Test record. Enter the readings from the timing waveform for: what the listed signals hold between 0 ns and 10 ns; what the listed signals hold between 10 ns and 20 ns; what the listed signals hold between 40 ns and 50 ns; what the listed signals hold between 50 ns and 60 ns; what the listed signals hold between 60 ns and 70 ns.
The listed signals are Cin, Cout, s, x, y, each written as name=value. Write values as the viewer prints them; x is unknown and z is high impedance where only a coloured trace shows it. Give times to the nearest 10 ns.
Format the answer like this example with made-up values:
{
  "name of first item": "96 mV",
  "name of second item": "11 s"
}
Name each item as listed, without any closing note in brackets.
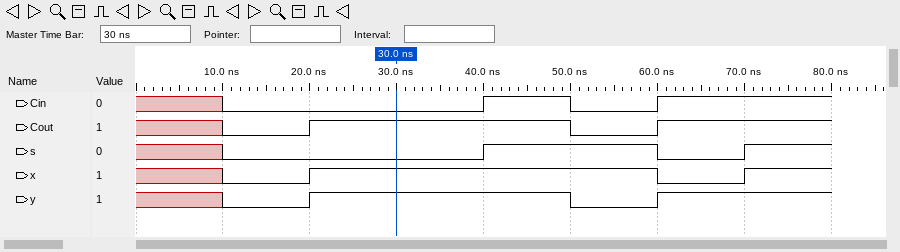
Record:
{
  "what the listed signals hold between 0 ns and 10 ns": "Cin=x, Cout=x, s=x, x=x, y=x",
  "what the listed signals hold between 10 ns and 20 ns": "Cin=0, Cout=0, s=0, x=0, y=0",
  "what the listed signals hold between 40 ns and 50 ns": "Cin=1, Cout=1, s=1, x=1, y=1",
  "what the listed signals hold between 50 ns and 60 ns": "Cin=0, Cout=0, s=1, x=1, y=0",
  "what the listed signals hold between 60 ns and 70 ns": "Cin=1, Cout=1, s=0, x=0, y=1"
}
